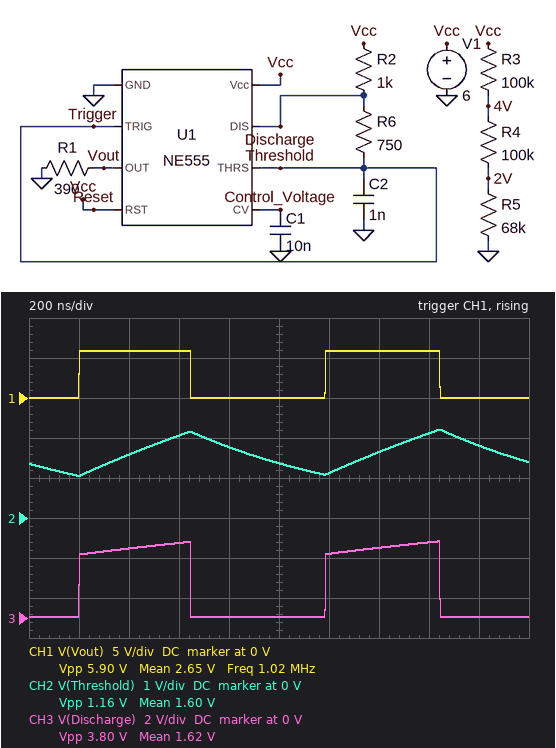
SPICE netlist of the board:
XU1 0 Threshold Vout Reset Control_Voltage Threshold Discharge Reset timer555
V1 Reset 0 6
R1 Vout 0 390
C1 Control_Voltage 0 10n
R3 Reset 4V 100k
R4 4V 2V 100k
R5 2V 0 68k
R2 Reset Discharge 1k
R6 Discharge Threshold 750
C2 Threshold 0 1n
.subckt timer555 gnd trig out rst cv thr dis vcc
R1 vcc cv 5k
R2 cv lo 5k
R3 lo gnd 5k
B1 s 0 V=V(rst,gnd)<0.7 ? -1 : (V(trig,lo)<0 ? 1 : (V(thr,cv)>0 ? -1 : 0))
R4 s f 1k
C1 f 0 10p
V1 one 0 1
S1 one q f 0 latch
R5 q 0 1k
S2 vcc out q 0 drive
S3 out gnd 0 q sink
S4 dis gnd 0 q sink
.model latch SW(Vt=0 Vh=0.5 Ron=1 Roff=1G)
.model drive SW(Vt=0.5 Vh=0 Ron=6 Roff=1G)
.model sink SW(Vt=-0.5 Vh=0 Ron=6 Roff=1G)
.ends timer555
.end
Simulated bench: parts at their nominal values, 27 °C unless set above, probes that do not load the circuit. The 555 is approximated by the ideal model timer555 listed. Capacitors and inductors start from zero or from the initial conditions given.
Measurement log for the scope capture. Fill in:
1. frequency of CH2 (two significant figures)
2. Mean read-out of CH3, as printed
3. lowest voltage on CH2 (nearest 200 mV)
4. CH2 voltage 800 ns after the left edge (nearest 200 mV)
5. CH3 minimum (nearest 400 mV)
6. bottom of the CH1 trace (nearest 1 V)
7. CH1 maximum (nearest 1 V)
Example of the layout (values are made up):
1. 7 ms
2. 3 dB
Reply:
1. 1.0 MHz
2. 1.62 V
3. 1.0 V
4. 1.8 V
5. 0 V
6. 0 V
7. 6 V
